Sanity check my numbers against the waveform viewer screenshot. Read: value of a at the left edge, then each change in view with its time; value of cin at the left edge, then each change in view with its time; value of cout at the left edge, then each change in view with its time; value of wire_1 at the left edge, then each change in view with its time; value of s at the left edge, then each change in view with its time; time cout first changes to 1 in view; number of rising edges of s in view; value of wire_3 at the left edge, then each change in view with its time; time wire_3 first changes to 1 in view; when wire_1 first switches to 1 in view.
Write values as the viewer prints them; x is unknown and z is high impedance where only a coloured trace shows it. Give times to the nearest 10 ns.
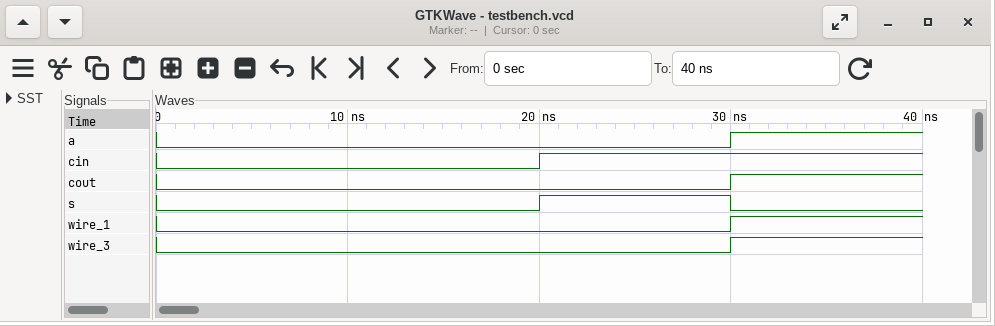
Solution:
0, 1 at 30 ns
0, 1 at 20 ns
0, 1 at 30 ns
0, 1 at 30 ns
0, 1 at 20 ns, 0 at 30 ns
30 ns
1
0, 1 at 30 ns
30 ns
30 ns
